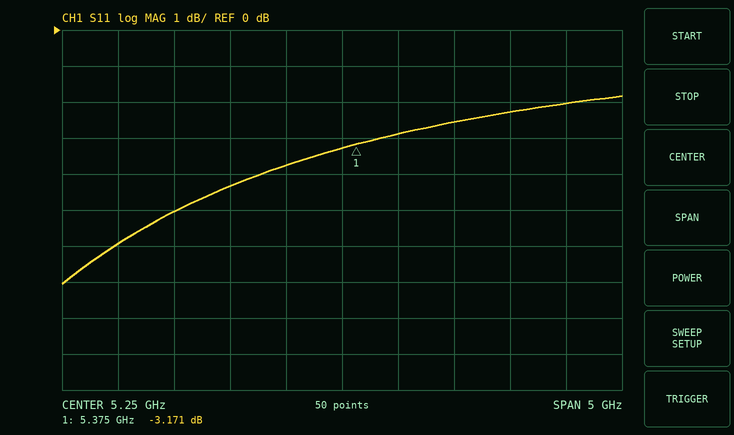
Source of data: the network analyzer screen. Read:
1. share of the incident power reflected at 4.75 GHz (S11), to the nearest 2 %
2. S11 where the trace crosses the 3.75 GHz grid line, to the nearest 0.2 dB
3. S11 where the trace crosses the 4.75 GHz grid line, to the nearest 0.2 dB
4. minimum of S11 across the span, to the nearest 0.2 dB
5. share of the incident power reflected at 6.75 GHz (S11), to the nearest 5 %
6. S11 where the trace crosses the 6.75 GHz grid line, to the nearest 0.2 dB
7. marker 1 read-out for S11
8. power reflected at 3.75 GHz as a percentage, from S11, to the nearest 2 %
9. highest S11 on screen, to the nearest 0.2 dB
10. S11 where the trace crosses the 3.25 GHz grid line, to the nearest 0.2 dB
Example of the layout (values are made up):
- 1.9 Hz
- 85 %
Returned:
- 42 %
- -5.0 dB
- -3.8 dB
- -7.0 dB
- 60 %
- -2.2 dB
- -3.171 dB
- 32 %
- -1.8 dB
- -6.0 dB
